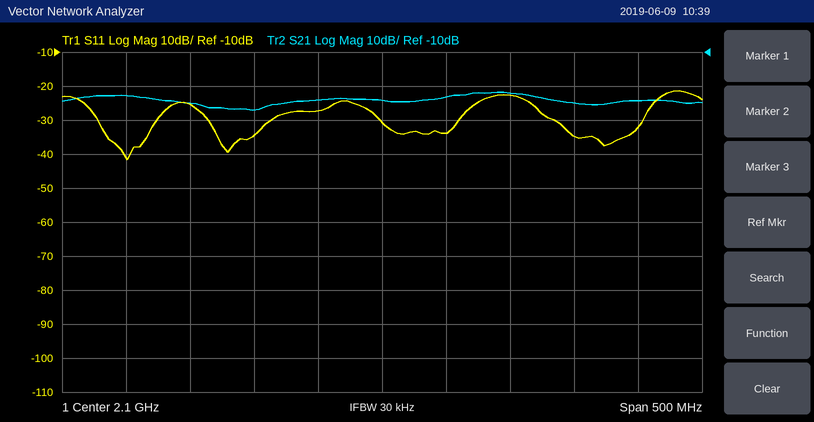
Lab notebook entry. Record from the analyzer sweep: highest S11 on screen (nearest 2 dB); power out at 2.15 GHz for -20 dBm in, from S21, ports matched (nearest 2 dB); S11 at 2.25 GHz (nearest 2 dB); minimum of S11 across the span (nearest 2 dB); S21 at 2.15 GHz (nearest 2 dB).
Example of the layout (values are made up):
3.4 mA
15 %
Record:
-22 dB
-44 dBm
-34 dB
-42 dB
-24 dB
